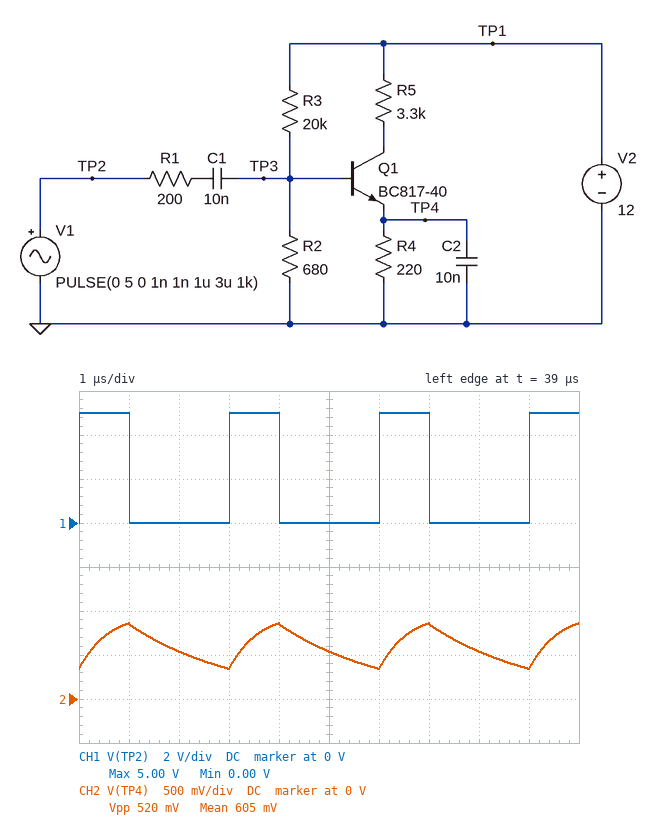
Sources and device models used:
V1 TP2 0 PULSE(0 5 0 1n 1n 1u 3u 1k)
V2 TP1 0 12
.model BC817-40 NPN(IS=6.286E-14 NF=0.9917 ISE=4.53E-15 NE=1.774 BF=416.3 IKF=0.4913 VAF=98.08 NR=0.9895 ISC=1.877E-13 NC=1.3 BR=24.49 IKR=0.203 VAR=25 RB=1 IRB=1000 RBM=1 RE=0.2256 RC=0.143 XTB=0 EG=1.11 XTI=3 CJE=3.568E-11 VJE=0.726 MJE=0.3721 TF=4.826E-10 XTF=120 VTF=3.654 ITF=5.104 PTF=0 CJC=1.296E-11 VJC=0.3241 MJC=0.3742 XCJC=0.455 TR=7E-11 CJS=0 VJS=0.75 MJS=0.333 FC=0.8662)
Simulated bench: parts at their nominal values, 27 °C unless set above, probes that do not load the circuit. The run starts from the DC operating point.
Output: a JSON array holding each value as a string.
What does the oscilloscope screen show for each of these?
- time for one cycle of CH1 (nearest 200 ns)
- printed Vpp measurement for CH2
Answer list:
["3.0 µs", "520 mV"]
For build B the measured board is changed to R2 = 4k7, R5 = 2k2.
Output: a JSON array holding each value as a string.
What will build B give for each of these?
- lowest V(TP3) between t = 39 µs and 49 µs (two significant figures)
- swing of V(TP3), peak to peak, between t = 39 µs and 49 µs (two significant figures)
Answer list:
["-2.9 V", "4.4 V"]
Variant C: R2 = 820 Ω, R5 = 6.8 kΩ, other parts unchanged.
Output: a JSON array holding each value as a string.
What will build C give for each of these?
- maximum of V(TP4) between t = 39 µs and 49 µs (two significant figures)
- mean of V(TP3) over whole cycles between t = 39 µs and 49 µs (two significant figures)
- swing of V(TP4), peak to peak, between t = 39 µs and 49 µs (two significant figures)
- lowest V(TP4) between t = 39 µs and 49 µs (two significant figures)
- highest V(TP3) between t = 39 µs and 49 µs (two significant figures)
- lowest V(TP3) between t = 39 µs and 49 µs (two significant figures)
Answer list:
["700 mV", "-800 mV", "420 mV", "280 mV", "1.4 V", "-2.1 V"]
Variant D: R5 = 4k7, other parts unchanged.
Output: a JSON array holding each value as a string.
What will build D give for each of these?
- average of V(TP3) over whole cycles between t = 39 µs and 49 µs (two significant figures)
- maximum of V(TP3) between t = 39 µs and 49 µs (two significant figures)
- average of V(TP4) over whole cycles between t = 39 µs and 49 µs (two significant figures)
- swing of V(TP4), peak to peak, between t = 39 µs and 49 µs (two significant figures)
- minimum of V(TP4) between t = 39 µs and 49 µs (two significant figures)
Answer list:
["-660 mV", "1.5 V", "540 mV", "470 mV", "310 mV"]
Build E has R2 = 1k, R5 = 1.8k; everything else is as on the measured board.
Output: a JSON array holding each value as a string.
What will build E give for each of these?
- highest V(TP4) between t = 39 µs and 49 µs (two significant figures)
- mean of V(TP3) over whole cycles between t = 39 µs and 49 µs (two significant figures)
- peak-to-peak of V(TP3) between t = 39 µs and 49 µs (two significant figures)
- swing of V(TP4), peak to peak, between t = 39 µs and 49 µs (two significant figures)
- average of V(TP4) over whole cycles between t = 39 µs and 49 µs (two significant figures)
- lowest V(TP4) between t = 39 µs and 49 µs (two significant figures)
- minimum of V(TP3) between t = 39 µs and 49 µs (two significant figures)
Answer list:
["1.1 V", "-690 mV", "3.8 V", "650 mV", "750 mV", "430 mV", "-2.0 V"]
